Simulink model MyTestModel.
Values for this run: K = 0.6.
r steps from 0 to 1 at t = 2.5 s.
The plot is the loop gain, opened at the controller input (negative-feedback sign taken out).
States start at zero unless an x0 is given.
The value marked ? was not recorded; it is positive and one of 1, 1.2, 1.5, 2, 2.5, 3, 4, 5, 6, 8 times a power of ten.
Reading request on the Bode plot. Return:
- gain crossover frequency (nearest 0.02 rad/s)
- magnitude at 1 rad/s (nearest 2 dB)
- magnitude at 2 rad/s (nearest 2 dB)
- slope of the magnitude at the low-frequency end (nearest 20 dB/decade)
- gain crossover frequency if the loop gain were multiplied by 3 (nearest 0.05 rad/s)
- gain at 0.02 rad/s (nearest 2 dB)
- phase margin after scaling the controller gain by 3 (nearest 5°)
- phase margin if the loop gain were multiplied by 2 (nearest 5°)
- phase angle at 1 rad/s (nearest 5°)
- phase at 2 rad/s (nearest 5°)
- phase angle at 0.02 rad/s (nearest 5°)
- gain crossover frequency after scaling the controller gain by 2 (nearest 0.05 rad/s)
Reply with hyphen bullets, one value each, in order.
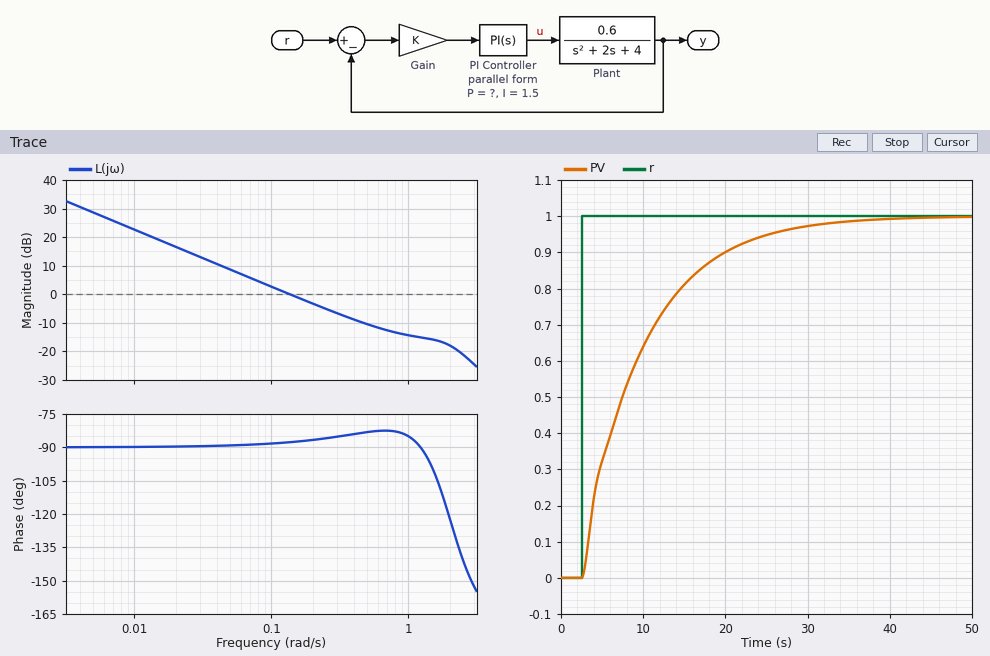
- 0.14 rad/s
- -14 dB
- -18 dB
- -20 dB/decade
- 0.45 rad/s
- 16 dB
- 95°
- 95°
- -85°
- -120°
- -90°
- 0.30 rad/s
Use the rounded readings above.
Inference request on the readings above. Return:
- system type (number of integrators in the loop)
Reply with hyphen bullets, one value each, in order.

- 1
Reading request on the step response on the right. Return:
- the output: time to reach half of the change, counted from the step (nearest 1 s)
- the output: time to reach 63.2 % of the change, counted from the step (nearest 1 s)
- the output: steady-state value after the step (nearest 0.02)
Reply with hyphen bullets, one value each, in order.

- 5 s
- 7 s
- 1.00
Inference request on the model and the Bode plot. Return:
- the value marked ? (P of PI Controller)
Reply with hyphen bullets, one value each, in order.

- 1.2
